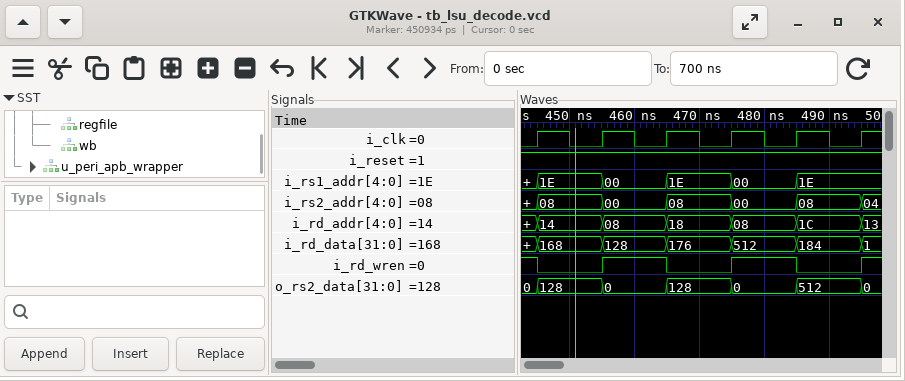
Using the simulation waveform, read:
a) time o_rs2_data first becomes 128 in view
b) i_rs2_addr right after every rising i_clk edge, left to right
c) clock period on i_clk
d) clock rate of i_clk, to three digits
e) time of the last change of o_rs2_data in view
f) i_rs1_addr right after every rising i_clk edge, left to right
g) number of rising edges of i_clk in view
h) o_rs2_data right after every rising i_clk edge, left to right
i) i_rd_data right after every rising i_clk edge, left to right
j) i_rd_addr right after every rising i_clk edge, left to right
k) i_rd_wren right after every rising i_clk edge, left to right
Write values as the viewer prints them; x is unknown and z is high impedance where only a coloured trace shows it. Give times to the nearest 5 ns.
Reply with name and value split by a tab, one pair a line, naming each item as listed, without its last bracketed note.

time o_rs2_data first becomes 128 in view	445 ns
i_rs2_addr right after every rising i_clk edge, left to right	08, 00, 08, 00, 08, 04
clock period on i_clk	10 ns
clock rate of i_clk, to three digits	100 MHz
time of the last change of o_rs2_data in view	495 ns
i_rs1_addr right after every rising i_clk edge, left to right	1E, 00, 1E, 00, 1E, 1E
number of rising edges of i_clk in view	6
o_rs2_data right after every rising i_clk edge, left to right	128, 0, 128, 0, 512, 0
i_rd_data right after every rising i_clk edge, left to right	168, 128, 176, 512, 184, 1
i_rd_addr right after every rising i_clk edge, left to right	14, 08, 18, 08, 1C, 13
i_rd_wren right after every rising i_clk edge, left to right	0 1 0 1 0 1
